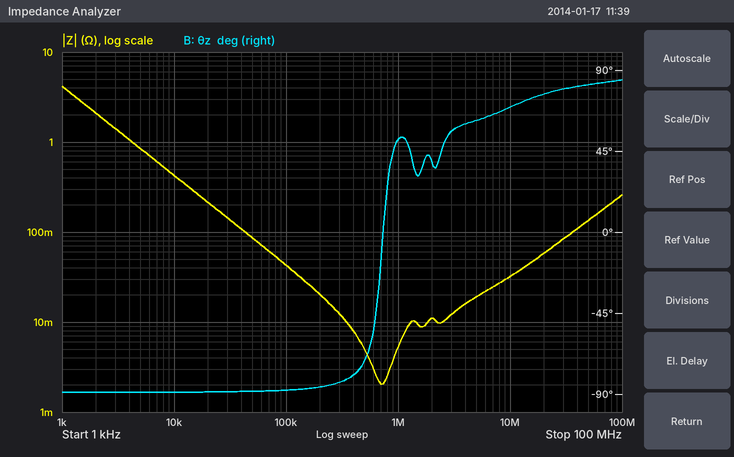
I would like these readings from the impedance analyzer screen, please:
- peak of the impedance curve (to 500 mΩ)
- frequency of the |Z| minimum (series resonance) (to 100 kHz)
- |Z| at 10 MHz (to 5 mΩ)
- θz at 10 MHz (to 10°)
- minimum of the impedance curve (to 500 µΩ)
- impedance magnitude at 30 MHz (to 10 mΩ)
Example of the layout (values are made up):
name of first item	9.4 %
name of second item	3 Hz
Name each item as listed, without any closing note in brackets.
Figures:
peak of the impedance curve	4.0 Ω
frequency of the |Z| minimum (series resonance)	700 kHz
|Z| at 10 MHz	30 mΩ
θz at 10 MHz	70°
minimum of the impedance curve	2.0 mΩ
impedance magnitude at 30 MHz	80 mΩ
